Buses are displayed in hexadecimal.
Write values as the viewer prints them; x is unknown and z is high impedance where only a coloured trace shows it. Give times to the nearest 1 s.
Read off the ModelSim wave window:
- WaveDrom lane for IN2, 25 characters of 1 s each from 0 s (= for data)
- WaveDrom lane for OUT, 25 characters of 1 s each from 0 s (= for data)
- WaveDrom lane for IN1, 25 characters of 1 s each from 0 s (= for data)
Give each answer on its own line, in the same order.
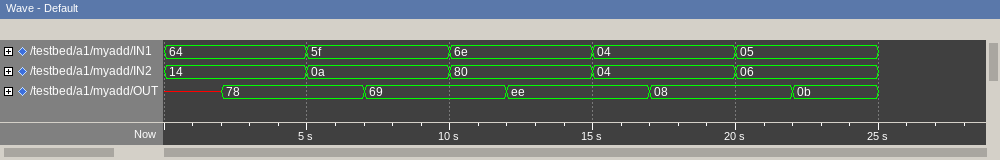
{name: 'IN2', wave: '=....=....=....=....=....', data: '14 0a 80 04 06'}
{name: 'OUT', wave: 'x.=....=....=....=....=..', data: '78 69 ee 08 0b'}
{name: 'IN1', wave: '=....=....=....=....=....', data: '64 5f 6e 04 05'}
